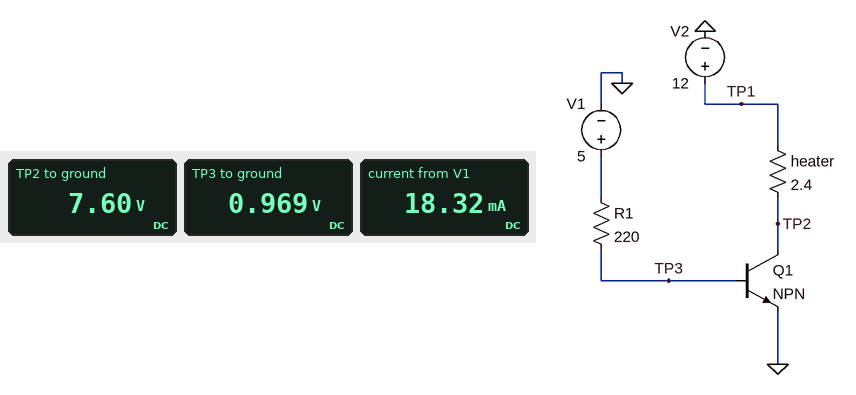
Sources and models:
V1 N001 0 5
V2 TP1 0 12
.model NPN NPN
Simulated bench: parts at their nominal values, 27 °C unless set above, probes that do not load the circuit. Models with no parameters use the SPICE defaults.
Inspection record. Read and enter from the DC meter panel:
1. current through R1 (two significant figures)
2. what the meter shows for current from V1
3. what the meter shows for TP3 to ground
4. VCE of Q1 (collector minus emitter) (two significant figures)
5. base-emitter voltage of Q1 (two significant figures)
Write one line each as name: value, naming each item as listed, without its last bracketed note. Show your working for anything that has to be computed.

current through R1: (5 V - 969 mV) / 220 Ω = 18 mA
what the meter shows for current from V1: 18.32 mA
what the meter shows for TP3 to ground: 0.969 V
VCE of Q1 (collector minus emitter): 7.6 V = 7.6 V
base-emitter voltage of Q1: 969 mV = 970 mV
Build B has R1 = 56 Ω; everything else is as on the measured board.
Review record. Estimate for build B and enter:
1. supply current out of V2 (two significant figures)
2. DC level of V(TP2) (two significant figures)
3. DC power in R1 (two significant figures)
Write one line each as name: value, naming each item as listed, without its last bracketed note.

supply current out of V2: 4.9 A
DC level of V(TP2): 140 mV
DC power in R1: 290 mW
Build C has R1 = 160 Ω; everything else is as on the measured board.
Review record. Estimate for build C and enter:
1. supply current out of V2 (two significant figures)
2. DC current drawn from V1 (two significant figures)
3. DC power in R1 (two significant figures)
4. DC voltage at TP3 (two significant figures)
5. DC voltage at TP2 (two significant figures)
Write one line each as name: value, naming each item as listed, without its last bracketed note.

supply current out of V2: 2.5 A
DC current drawn from V1: 25 mA
DC power in R1: 100 mW
DC voltage at TP3: 980 mV
DC voltage at TP2: 6.0 V
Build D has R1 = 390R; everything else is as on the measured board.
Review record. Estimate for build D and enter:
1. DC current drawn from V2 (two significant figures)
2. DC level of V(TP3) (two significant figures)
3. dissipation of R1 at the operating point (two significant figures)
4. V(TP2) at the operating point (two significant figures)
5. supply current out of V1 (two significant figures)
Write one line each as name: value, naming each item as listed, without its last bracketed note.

DC current drawn from V2: 1.0 A
DC level of V(TP3): 950 mV
dissipation of R1 at the operating point: 42 mW
V(TP2) at the operating point: 9.5 V
supply current out of V1: 10 mA
